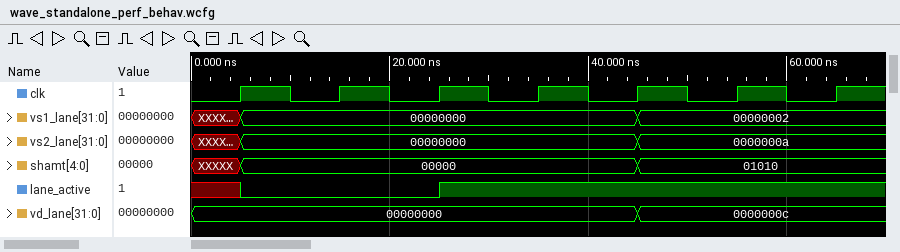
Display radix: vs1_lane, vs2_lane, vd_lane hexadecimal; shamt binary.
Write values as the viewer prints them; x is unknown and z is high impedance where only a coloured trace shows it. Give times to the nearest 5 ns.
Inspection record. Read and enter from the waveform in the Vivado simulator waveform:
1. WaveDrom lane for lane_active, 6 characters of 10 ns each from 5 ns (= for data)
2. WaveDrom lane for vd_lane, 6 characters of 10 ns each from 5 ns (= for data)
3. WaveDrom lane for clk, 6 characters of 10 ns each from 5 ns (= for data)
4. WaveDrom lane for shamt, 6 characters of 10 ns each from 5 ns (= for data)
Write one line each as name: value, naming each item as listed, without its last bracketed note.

WaveDrom lane for lane_active, 6 characters of 10 ns each from 5 ns: {name: 'lane_active', wave: '0.1...'}
WaveDrom lane for vd_lane, 6 characters of 10 ns each from 5 ns: {name: 'vd_lane', wave: '=...=.', data: '00000000 0000000c'}
WaveDrom lane for clk, 6 characters of 10 ns each from 5 ns: {name: 'clk', wave: 'p.....'}
WaveDrom lane for shamt, 6 characters of 10 ns each from 5 ns: {name: 'shamt', wave: '=...=.', data: '00000 01010'}
